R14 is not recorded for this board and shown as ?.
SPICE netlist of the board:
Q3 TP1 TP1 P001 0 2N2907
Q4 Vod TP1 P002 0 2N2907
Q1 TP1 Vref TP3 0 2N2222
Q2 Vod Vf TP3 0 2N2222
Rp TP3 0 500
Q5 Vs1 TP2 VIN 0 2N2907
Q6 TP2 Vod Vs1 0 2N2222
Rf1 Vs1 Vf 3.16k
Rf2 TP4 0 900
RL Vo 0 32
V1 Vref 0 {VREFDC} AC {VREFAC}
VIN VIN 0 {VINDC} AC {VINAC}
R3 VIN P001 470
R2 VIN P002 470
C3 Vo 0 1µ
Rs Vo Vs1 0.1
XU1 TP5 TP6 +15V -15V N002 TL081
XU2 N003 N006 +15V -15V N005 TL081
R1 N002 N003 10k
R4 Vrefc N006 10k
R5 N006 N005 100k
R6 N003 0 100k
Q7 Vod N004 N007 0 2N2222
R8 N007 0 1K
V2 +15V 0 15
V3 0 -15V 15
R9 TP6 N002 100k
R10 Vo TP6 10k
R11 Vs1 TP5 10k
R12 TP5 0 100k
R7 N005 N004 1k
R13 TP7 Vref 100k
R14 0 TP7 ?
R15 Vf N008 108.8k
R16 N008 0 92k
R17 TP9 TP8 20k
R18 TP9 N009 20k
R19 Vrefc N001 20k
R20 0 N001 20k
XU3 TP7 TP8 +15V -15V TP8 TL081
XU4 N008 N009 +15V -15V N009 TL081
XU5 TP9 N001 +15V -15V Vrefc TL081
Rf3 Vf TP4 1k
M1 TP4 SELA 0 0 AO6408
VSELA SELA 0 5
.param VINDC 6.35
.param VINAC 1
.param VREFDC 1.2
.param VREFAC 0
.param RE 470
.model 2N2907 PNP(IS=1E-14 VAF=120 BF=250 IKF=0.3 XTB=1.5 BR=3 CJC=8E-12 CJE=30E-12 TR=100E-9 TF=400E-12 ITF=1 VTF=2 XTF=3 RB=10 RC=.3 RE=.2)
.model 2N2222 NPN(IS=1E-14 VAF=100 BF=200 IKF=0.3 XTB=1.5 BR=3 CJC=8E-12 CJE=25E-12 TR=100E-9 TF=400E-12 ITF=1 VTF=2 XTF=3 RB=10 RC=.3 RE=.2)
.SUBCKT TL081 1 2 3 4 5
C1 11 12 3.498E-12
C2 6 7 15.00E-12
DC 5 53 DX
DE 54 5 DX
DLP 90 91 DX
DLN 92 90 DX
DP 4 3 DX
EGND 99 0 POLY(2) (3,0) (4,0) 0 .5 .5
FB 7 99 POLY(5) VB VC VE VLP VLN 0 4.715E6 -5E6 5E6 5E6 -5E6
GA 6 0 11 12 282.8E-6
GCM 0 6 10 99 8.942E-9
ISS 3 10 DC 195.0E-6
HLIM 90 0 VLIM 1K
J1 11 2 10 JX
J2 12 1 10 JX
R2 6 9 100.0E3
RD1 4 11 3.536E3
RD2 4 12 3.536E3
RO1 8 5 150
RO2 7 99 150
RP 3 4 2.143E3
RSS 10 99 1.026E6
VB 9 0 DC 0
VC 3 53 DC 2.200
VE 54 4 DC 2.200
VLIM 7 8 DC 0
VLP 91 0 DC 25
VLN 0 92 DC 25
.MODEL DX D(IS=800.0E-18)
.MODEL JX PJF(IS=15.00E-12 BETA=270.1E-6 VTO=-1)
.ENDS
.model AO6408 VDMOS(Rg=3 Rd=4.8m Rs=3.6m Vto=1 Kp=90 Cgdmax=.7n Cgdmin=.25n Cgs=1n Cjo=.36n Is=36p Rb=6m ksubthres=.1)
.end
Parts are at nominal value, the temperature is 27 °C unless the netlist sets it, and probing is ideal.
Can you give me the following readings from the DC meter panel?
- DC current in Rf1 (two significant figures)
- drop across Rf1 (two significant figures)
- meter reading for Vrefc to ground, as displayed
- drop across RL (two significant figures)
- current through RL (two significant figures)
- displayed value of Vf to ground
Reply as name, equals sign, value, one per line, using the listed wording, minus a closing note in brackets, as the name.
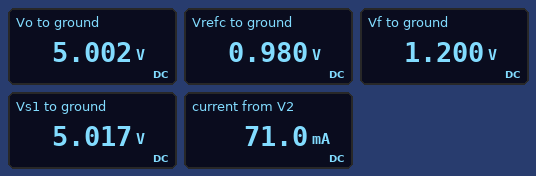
DC current in Rf1 = 1.2 mA
drop across Rf1 = 3.8 V
meter reading for Vrefc to ground, as displayed = 0.980 V
drop across RL = 5.0 V
current through RL = 160 mA
displayed value of Vf to ground = 1.200 V
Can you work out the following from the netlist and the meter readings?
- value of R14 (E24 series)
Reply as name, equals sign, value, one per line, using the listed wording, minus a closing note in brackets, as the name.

value of R14 = 56 kΩ
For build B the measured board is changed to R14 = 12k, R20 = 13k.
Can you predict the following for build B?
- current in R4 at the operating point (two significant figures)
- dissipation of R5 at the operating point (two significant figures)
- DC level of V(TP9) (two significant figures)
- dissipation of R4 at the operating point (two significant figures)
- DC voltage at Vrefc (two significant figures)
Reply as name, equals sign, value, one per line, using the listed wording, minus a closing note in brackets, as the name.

current in R4 at the operating point = 72 µA
dissipation of R5 at the operating point = 520 µW
DC level of V(TP9) = 340 mV
dissipation of R4 at the operating point = 52 µW
DC voltage at Vrefc = 860 mV
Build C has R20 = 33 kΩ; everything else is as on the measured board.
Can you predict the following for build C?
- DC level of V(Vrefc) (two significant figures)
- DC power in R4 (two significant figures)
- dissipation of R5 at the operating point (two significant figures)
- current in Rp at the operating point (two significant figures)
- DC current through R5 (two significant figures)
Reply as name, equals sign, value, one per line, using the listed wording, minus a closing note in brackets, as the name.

DC level of V(Vrefc) = 790 mV
DC power in R4 = 42 µW
dissipation of R5 at the operating point = 420 µW
current in Rp at the operating point = 1.1 mA
DC current through R5 = 65 µA
